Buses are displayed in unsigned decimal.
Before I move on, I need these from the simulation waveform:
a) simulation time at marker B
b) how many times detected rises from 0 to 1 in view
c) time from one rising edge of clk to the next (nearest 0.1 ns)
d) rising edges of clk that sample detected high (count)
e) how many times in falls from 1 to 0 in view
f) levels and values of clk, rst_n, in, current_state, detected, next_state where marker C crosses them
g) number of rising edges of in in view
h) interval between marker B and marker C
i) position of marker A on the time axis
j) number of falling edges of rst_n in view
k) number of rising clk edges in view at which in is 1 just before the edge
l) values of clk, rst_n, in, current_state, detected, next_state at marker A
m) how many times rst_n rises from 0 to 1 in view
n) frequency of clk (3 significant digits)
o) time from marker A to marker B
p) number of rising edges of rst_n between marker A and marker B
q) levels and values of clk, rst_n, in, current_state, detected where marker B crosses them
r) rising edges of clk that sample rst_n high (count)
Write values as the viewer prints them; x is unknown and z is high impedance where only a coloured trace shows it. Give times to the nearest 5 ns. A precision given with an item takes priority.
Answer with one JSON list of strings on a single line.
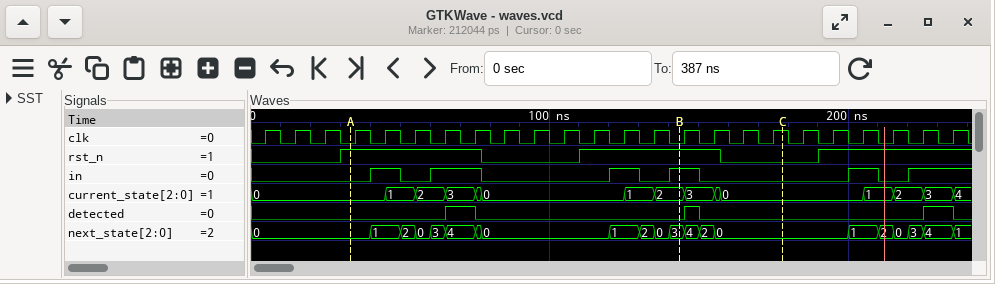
["145 ns", "3", "10 ns", "2", "5", "clk=1, rst_n=0, in=0, current_state=0, detected=0, next_state=0", "6", "35 ns", "35 ns", "2", "8", "clk=0, rst_n=1, in=0, current_state=0, detected=0, next_state=0", "3", "100 MHz", "110 ns", "1", "clk=0, rst_n=1, in=1, current_state=2, detected=0", "15"]
